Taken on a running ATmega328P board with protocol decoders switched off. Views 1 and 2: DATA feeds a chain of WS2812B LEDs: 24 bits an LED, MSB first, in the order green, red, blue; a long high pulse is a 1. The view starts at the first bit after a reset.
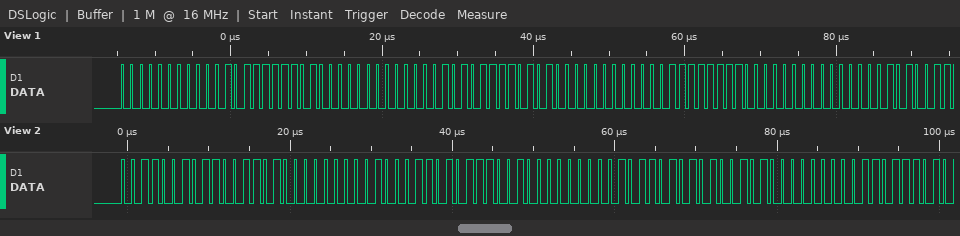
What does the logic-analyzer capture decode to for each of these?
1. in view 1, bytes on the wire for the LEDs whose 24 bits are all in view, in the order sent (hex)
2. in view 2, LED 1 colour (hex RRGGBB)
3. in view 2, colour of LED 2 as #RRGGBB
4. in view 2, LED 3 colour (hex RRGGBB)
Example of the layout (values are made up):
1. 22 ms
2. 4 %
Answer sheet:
1. 00 17 E8 00 2B D4 00 3F C0
2. #CD3200
3. #B94600
4. #A55A00
